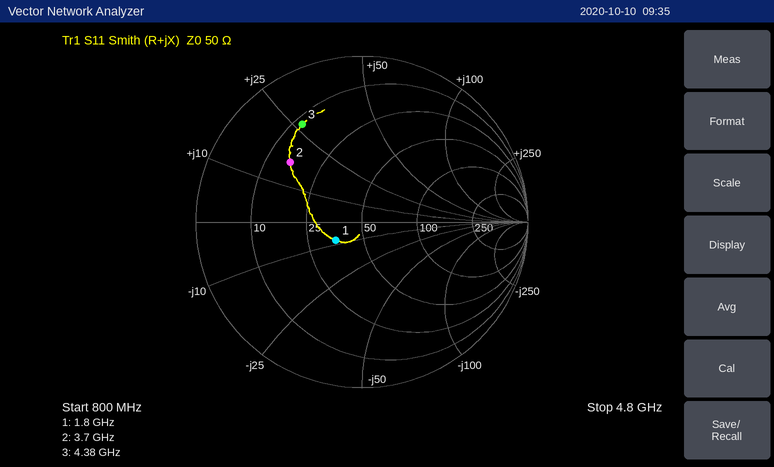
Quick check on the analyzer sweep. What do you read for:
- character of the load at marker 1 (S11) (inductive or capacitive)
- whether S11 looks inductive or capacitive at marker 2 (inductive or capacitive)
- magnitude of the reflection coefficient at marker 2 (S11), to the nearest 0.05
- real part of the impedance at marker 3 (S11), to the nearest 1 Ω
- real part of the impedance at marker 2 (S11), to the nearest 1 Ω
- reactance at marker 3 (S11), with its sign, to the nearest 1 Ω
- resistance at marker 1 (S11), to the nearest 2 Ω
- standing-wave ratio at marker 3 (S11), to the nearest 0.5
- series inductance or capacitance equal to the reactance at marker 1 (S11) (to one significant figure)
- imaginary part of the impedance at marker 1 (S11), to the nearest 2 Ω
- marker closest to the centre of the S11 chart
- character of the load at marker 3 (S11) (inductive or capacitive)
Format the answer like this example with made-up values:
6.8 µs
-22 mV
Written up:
capacitive
inductive
0.55
12 Ω
16 Ω
+27 Ω
36 Ω
5.5
10 pF
-8 Ω
marker 1
inductive
